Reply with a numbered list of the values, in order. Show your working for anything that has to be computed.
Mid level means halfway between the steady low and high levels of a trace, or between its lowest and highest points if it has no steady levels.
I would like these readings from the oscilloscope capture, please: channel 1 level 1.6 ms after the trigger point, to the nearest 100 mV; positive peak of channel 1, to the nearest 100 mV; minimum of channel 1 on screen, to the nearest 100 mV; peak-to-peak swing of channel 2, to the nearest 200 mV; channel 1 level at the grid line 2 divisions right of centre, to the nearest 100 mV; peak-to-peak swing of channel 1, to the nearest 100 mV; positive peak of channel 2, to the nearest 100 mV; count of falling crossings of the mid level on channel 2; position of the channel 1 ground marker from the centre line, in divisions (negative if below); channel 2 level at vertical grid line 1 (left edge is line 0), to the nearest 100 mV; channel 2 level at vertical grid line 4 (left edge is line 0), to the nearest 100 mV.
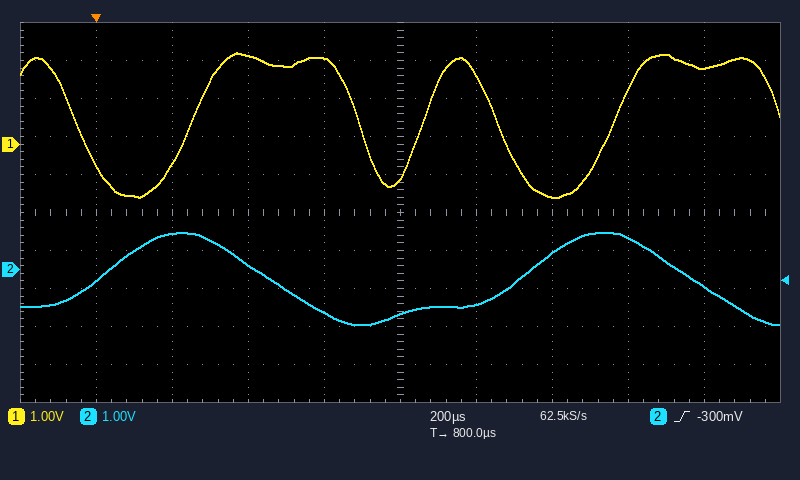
1. 2.0 V
2. 2.4 V
3. -1.4 V
4. 2.4 V
5. -1.4 V
6. 2.4 V − (-1.4 V) = 3.8 V
7. 1.0 V
8. 2
9. +1.8 div
10. -300 mV
11. -1.1 V
